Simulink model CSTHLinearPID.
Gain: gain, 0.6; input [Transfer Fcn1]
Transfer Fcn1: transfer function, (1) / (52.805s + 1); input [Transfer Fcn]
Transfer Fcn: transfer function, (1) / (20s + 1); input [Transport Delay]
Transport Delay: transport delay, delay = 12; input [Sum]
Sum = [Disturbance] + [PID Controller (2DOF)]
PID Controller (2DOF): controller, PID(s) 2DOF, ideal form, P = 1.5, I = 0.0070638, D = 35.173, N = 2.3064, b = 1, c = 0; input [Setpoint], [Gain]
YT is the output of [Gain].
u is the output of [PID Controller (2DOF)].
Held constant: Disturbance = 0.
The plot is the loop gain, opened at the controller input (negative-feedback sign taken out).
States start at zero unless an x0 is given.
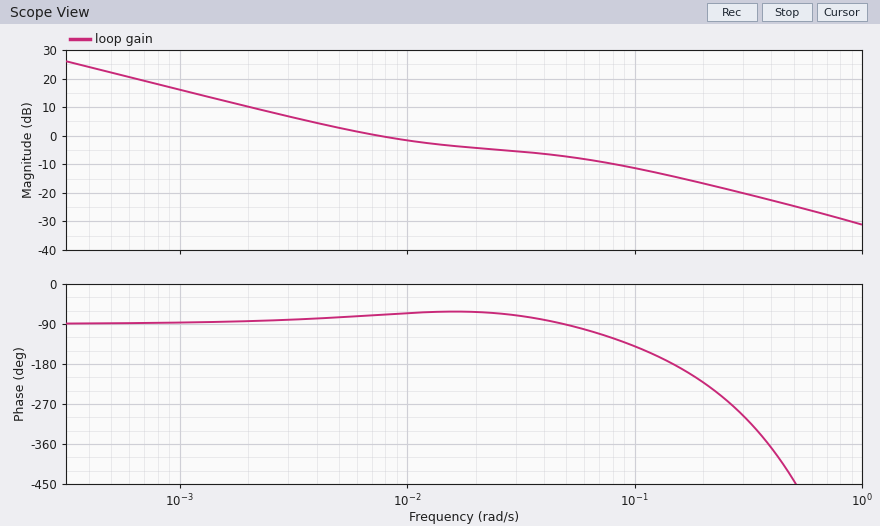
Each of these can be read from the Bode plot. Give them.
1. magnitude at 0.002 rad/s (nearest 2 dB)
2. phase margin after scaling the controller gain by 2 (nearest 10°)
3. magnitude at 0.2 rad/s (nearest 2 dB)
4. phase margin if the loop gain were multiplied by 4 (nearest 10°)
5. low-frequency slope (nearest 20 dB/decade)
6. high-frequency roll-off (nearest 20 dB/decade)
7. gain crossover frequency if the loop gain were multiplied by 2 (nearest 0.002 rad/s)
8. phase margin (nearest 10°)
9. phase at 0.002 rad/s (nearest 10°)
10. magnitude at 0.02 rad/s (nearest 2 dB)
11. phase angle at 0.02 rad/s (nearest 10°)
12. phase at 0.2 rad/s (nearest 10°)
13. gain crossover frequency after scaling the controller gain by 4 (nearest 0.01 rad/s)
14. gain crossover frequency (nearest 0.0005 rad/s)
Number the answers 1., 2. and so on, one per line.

1. 10 dB
2. 100°
3. -16 dB
4. 30°
5. -20 dB/decade
6. -20 dB/decade
7. 0.036 rad/s
8. 110°
9. -80°
10. -4 dB
11. -60°
12. -220°
13. 0.11 rad/s
14. 0.0075 rad/s
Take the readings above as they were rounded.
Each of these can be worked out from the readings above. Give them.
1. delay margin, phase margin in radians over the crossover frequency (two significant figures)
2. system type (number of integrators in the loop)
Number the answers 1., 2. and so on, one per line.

1. 260 s
2. 1
